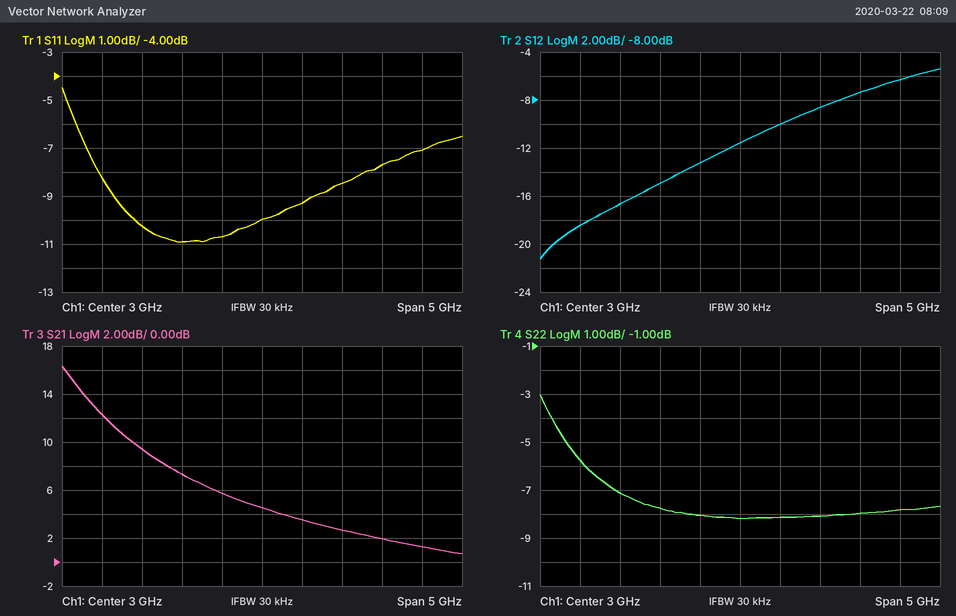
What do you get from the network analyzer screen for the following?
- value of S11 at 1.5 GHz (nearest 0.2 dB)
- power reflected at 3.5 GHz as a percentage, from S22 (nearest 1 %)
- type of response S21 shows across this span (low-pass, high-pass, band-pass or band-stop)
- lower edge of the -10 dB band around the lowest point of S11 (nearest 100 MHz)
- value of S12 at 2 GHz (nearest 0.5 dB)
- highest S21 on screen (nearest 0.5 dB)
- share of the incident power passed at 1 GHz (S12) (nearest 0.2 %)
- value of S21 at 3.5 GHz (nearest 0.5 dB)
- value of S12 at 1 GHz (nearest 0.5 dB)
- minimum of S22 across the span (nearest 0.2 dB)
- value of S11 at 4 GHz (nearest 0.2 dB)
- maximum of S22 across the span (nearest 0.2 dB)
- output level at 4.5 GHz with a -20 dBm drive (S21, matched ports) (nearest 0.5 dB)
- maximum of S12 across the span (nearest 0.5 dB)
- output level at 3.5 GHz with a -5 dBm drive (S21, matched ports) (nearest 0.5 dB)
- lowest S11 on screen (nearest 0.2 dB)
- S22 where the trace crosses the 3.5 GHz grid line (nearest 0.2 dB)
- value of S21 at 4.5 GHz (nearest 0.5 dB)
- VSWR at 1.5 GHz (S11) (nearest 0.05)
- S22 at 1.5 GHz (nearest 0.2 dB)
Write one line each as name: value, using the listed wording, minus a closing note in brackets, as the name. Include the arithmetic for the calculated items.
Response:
value of S11 at 1.5 GHz: -10.2 dB
power reflected at 3.5 GHz as a percentage, from S22: 10^(-8.2/10) ≈ 15 %
type of response S21 shows across this span: low-pass
lower edge of the -10 dB band around the lowest point of S11: 1.4 GHz
value of S12 at 2 GHz: -15.0 dB
highest S21 on screen: 16.5 dB
share of the incident power passed at 1 GHz (S12): 10^(-18.5/10) ≈ 1.4 %
value of S21 at 3.5 GHz: 3.5 dB
value of S12 at 1 GHz: -18.5 dB
minimum of S22 across the span: -8.2 dB
value of S11 at 4 GHz: -8.4 dB
maximum of S22 across the span: -3.0 dB
output level at 4.5 GHz with a -20 dBm drive (S21, matched ports): -20 dBm + (2.0 dB) = -18.0 dBm
maximum of S12 across the span: -5.5 dB
output level at 3.5 GHz with a -5 dBm drive (S21, matched ports): -5 dBm + (3.5 dB) = -1.5 dBm
lowest S11 on screen: -11.0 dB
S22 where the trace crosses the 3.5 GHz grid line: -8.2 dB
value of S21 at 4.5 GHz: 2.0 dB
VSWR at 1.5 GHz (S11): |Γ| = 10^(-10.2/20) = 0.3090; VSWR = (1 + 0.3090)/(1 − 0.3090) ≈ 1.89, so 1.90 to the nearest 0.05
S22 at 1.5 GHz: -7.2 dB
